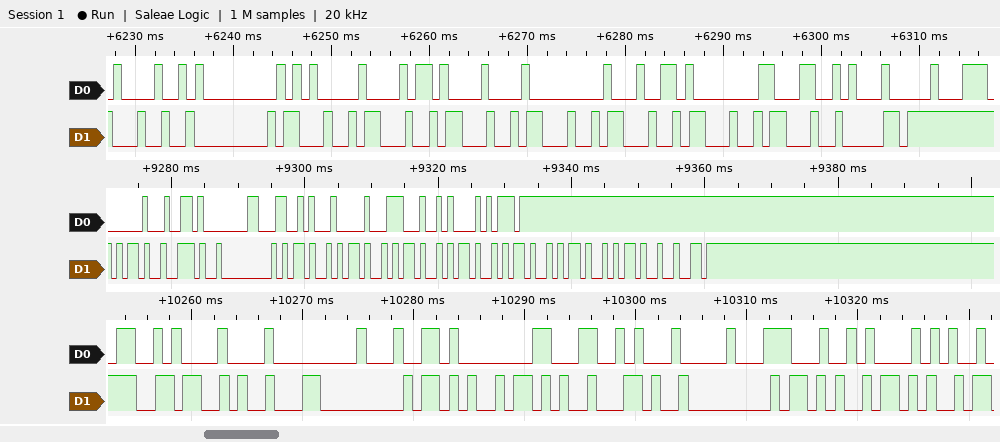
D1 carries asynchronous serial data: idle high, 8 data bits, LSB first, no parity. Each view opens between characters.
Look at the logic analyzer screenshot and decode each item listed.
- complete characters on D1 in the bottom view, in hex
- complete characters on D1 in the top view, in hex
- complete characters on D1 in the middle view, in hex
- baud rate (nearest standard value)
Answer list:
36, 89, 00, 2B, 2B, 2C, 00, 2B, 2B
24, 00, 23, 23, 23, 23, 23, 23, 23, B0
2D, 2E, 00, 2D, 2D, 2D, 2D, 2D, 2D, 2D, B2
1200 baud
